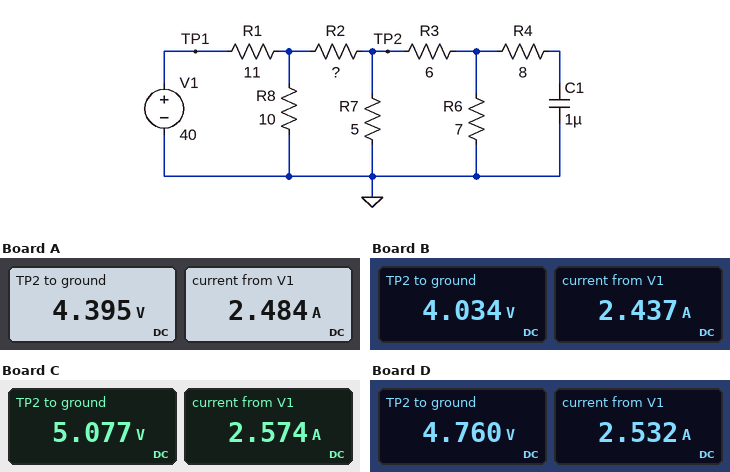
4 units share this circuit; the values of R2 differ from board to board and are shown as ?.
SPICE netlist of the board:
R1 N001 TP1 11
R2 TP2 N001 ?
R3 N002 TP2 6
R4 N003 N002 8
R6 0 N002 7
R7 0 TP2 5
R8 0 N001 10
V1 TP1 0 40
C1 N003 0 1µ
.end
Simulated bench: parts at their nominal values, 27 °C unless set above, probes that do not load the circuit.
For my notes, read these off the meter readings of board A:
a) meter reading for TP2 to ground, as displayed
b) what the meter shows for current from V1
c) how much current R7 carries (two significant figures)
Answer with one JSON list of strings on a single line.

["4.395 V", "2.484 A", "880 mA"]
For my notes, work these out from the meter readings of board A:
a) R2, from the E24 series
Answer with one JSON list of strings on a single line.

["6.8 Ω"]
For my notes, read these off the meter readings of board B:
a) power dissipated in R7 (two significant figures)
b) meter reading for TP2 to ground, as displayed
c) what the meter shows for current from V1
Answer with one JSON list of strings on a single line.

["3.3 W", "4.034 V", "2.437 A"]
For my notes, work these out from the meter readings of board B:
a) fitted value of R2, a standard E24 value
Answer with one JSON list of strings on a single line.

["8.2 Ω"]
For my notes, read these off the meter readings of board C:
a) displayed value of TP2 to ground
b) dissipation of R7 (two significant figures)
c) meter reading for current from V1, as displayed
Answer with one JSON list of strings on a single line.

["5.077 V", "5.2 W", "2.574 A"]
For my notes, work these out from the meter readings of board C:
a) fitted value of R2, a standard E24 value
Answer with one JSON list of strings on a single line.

["4.7 Ω"]
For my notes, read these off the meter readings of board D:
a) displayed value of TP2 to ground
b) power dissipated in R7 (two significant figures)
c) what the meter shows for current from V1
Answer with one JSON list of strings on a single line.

["4.760 V", "4.5 W", "2.532 A"]
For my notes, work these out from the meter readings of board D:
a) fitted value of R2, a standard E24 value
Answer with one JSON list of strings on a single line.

["5.6 Ω"]
